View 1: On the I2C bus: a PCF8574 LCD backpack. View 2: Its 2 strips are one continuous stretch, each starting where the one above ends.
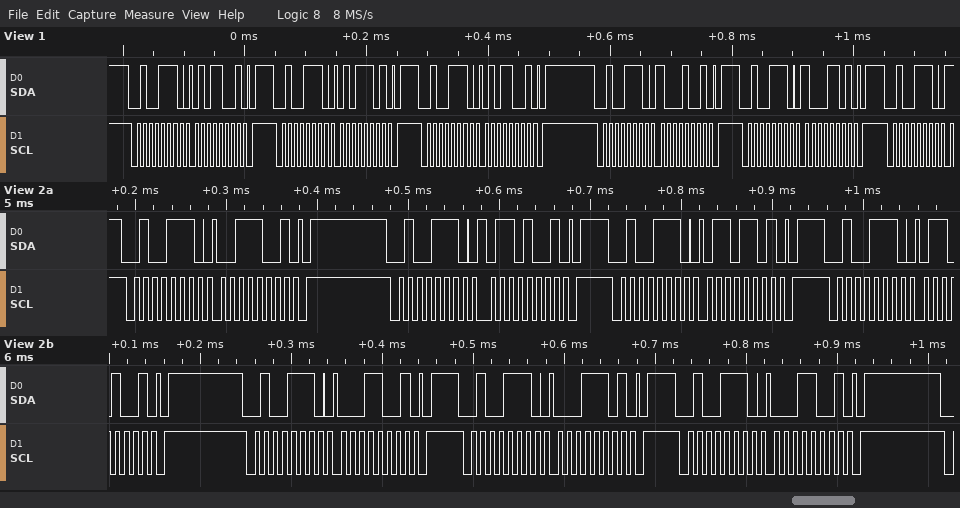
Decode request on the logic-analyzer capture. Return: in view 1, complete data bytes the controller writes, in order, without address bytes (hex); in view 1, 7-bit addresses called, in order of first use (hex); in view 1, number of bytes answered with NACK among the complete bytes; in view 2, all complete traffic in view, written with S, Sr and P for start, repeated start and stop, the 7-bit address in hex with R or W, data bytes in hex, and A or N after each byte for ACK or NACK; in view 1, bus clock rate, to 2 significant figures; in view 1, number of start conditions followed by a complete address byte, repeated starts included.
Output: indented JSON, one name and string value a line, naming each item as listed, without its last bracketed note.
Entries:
{
  "in view 1, complete data bytes the controller writes, in order, without address bytes": "59 5D 59 89 8D",
  "in view 1, 7-bit addresses called, in order of first use": "0x27",
  "in view 1, number of bytes answered with NACK among the complete bytes": "0",
  "in view 2, all complete traffic in view, written with S, Sr and P for start, repeated start and stop, the 7-bit address in hex with R or W, data bytes in hex, and A or N after each byte for ACK or NACK": "S 27W A 39 A P S 27W A 69 A P S 27W A 6D A P S 27W A 69 A P S 27W A 19 A P S 27W A 1D A P S 27W A 19 A P",
  "in view 1, bus clock rate, to 2 significant figures": "100 kHz",
  "in view 1, number of start conditions followed by a complete address byte, repeated starts included": "6"
}
